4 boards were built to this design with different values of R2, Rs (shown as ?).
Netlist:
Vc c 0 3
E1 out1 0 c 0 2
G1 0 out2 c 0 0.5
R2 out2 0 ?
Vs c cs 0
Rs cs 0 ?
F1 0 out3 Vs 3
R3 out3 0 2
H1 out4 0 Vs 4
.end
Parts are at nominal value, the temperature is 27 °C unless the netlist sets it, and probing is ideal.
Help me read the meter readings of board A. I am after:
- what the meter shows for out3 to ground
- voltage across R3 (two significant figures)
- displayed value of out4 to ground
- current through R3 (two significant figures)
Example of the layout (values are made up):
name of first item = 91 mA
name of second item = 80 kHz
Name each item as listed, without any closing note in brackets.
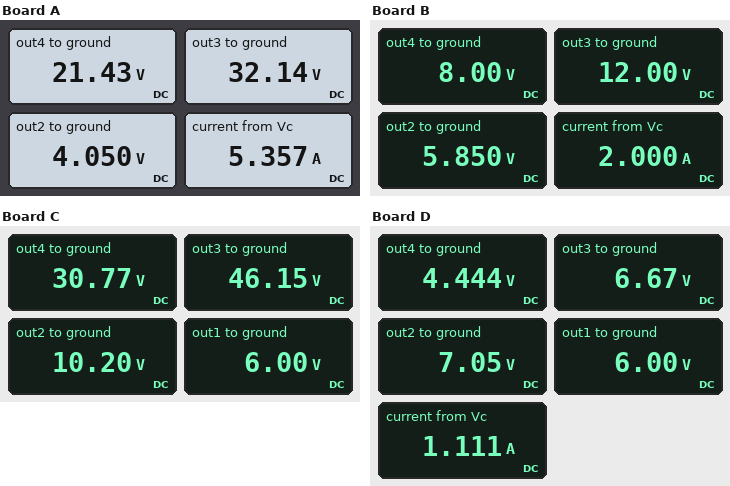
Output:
what the meter shows for out3 to ground = 32.14 V
voltage across R3 = 32 V
displayed value of out4 to ground = 21.43 V
current through R3 = 16 A
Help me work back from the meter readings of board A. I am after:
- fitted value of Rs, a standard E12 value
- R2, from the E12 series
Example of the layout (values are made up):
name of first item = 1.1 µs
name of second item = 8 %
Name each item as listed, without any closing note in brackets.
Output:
fitted value of Rs, a standard E12 value = 0.56 Ω
R2, from the E12 series = 2.7 Ω
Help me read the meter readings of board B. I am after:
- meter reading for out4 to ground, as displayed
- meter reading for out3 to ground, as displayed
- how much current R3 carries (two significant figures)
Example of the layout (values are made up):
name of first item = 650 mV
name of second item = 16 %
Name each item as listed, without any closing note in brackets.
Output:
meter reading for out4 to ground, as displayed = 8.00 V
meter reading for out3 to ground, as displayed = 12.00 V
how much current R3 carries = 6.0 A
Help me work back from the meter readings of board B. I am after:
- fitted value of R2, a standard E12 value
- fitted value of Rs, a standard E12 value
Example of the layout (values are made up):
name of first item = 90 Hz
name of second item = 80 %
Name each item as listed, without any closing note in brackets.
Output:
fitted value of R2, a standard E12 value = 3.9 Ω
fitted value of Rs, a standard E12 value = 1.5 Ω
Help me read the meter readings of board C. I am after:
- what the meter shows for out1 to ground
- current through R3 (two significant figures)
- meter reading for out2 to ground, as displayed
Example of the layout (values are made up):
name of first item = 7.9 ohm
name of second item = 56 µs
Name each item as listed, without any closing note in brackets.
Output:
what the meter shows for out1 to ground = 6.00 V
current through R3 = 23 A
meter reading for out2 to ground, as displayed = 10.20 V
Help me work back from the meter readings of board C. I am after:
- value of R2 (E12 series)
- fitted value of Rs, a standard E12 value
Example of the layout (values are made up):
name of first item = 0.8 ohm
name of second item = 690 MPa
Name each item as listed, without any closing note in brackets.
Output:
value of R2 = 6.8 Ω
fitted value of Rs, a standard E12 value = 0.39 Ω
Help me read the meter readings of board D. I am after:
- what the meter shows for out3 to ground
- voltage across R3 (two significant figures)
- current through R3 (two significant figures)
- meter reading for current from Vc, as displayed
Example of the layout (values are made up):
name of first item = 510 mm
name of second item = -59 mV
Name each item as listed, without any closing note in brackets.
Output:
what the meter shows for out3 to ground = 6.67 V
voltage across R3 = 6.7 V
current through R3 = 3.3 A
meter reading for current from Vc, as displayed = 1.111 A
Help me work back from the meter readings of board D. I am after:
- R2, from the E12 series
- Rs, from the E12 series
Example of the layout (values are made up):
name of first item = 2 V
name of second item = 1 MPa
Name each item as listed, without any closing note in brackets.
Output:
R2, from the E12 series = 4.7 Ω
Rs, from the E12 series = 2.7 Ω
